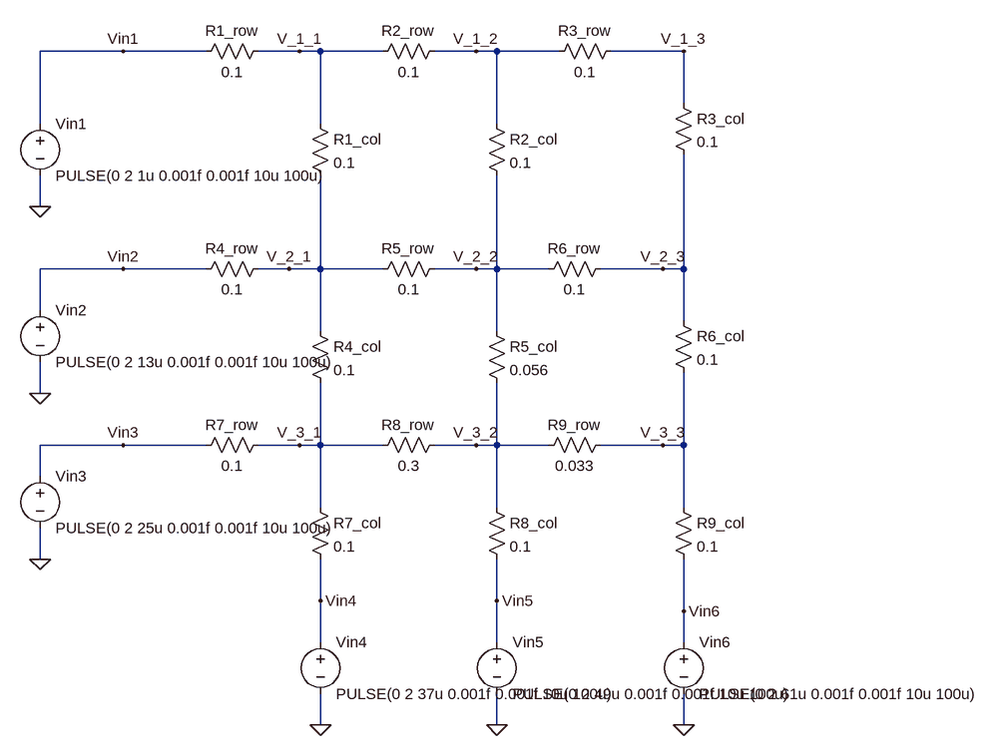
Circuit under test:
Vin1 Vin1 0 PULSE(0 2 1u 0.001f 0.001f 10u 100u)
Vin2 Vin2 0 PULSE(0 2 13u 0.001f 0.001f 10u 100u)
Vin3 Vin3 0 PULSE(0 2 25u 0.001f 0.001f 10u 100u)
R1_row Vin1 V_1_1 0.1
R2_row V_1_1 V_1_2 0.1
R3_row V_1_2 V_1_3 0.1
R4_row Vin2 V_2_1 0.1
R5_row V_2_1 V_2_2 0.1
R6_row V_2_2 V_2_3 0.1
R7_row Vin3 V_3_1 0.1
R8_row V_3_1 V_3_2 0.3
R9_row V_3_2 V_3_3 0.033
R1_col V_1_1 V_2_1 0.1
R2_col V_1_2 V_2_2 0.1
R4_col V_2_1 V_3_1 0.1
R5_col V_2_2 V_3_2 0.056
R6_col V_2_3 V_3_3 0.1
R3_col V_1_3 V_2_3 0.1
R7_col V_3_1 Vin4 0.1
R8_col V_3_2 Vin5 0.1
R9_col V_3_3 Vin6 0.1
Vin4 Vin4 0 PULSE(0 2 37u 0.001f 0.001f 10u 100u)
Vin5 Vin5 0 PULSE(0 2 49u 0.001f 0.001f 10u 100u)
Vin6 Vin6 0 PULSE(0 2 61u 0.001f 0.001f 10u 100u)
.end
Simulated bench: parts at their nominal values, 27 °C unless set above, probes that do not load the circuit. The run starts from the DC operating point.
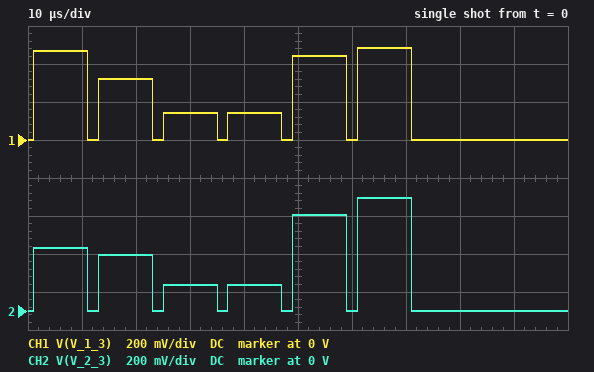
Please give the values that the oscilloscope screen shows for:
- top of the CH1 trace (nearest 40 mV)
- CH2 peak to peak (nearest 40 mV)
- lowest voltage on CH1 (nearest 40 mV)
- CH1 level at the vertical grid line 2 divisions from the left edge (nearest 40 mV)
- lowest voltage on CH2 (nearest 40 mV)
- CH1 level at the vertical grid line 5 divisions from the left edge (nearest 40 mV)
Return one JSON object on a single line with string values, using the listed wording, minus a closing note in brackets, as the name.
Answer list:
{"top of the CH1 trace": "480 mV", "CH2 peak to peak": "600 mV", "lowest voltage on CH1": "0 V", "CH1 level at the vertical grid line 2 divisions from the left edge": "320 mV", "lowest voltage on CH2": "0 V", "CH1 level at the vertical grid line 5 divisions from the left edge": "440 mV"}
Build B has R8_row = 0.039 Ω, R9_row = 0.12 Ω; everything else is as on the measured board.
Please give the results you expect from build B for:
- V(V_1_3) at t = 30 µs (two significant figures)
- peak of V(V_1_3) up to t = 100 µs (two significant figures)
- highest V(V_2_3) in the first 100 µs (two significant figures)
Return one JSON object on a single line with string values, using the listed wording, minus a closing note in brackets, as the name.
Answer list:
{"V(V_1_3) at t = 30 µs": "210 mV", "peak of V(V_1_3) up to t = 100 µs": "470 mV", "highest V(V_2_3) in the first 100 µs": "610 mV"}
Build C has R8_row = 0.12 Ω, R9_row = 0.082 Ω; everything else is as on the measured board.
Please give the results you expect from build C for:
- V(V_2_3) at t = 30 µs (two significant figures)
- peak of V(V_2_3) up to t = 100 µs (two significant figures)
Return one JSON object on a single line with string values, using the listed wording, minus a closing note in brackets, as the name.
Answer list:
{"V(V_2_3) at t = 30 µs": "170 mV", "peak of V(V_2_3) up to t = 100 µs": "610 mV"}
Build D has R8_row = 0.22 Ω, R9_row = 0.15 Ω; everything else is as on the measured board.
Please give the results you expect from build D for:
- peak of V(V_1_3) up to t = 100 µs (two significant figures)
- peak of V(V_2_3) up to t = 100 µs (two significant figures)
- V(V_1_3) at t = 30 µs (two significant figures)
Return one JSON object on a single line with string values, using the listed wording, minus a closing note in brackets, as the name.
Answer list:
{"peak of V(V_1_3) up to t = 100 µs": "510 mV", "peak of V(V_2_3) up to t = 100 µs": "660 mV", "V(V_1_3) at t = 30 µs": "150 mV"}
